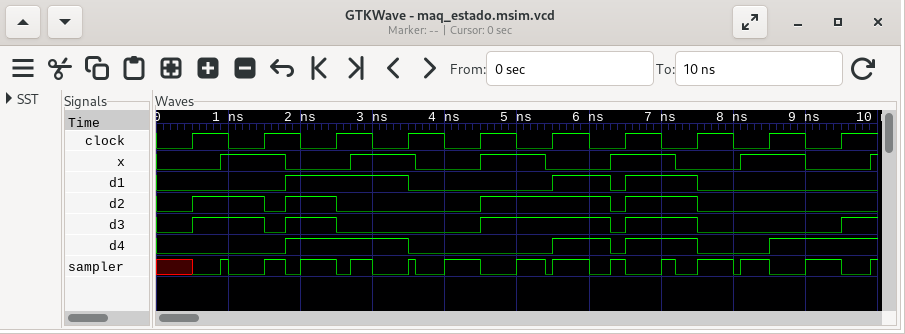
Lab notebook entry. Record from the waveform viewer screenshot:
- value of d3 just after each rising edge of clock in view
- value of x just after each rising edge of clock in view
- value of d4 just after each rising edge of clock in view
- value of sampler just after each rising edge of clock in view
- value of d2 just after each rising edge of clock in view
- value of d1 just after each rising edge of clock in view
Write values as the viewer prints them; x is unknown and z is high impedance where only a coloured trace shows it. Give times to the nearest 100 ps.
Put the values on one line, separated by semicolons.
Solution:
1 0 0 0 1 1 1 0 0 1; 0 1 0 1 1 0 1 0 1 0; 0 0 1 0 0 1 1 0 1 1; 0 1 0 1 0 1 0 1 0 0; 1 0 0 0 1 1 1 0 0 0; 0 0 1 0 0 1 1 0 0 0
